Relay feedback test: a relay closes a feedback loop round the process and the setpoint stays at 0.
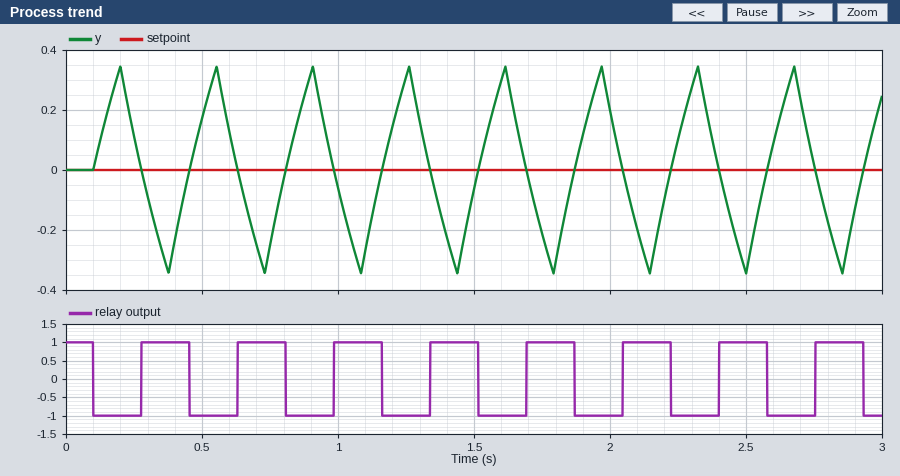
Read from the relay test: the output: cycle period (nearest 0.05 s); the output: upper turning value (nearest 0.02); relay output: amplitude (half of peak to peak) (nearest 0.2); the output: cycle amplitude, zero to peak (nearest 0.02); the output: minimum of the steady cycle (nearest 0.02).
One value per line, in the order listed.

0.35 s
0.34
1.0
0.34
-0.34
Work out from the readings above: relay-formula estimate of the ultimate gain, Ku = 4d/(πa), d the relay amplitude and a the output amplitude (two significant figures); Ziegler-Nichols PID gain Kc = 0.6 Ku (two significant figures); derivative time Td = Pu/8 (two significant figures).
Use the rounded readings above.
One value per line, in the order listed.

3.7
2.2
0.044 s
